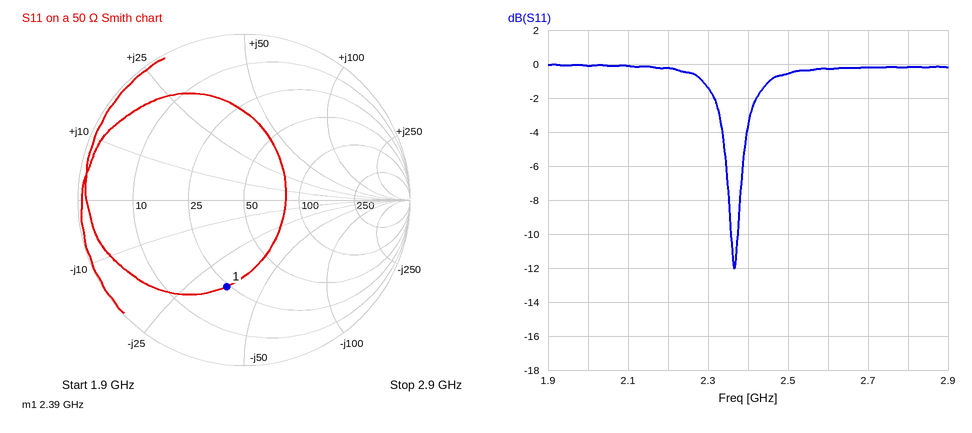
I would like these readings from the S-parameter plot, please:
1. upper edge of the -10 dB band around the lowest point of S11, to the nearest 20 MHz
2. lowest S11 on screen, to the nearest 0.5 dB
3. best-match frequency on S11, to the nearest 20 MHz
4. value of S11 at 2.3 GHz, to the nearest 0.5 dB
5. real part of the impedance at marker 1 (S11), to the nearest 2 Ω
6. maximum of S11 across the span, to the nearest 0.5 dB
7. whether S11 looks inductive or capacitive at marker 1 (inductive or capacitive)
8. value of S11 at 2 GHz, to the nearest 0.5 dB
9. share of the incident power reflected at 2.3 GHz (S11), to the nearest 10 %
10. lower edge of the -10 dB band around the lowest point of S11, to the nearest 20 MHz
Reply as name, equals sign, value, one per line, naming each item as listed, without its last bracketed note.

upper edge of the -10 dB band around the lowest point of S11, to the nearest 20 MHz = 2.38 GHz
lowest S11 on screen, to the nearest 0.5 dB = -12.0 dB
best-match frequency on S11, to the nearest 20 MHz = 2.36 GHz
value of S11 at 2.3 GHz, to the nearest 0.5 dB = -1.5 dB
real part of the impedance at marker 1 (S11), to the nearest 2 Ω = 24 Ω
maximum of S11 across the span, to the nearest 0.5 dB = 0.0 dB
whether S11 looks inductive or capacitive at marker 1 = capacitive
value of S11 at 2 GHz, to the nearest 0.5 dB = 0.0 dB
share of the incident power reflected at 2.3 GHz (S11), to the nearest 10 % = 70 %
lower edge of the -10 dB band around the lowest point of S11, to the nearest 20 MHz = 2.36 GHz
